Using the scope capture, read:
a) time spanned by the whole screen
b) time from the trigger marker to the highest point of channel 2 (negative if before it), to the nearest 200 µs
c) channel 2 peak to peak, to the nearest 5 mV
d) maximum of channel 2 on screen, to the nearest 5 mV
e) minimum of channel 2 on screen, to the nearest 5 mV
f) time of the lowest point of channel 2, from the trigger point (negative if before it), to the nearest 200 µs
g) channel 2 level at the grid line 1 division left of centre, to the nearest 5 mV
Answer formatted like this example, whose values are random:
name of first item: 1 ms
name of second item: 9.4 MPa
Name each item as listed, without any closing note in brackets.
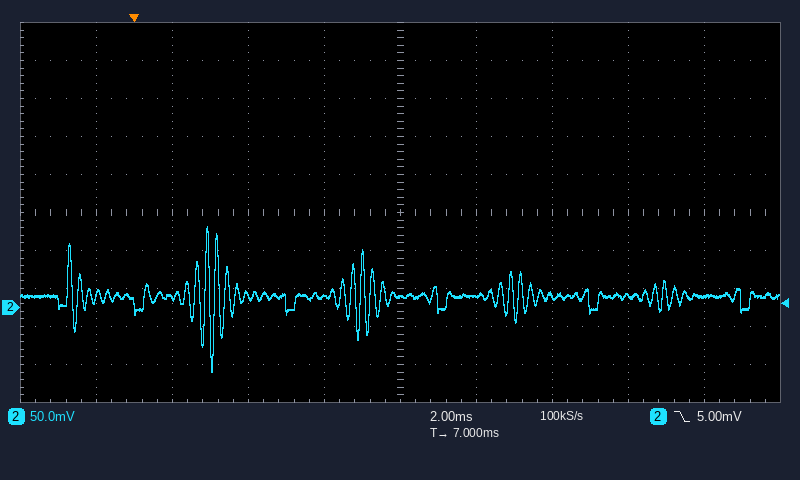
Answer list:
time spanned by the whole screen: 20 ms
time from the trigger marker to the highest point of channel 2 (negative if before it), to the nearest 200 µs: +2.0 ms
channel 2 peak to peak, to the nearest 5 mV: 190 mV
maximum of channel 2 on screen, to the nearest 5 mV: 105 mV
minimum of channel 2 on screen, to the nearest 5 mV: -85 mV
time of the lowest point of channel 2, from the trigger point (negative if before it), to the nearest 200 µs: +2.0 ms
channel 2 level at the grid line 1 division left of centre, to the nearest 5 mV: 15 mV
